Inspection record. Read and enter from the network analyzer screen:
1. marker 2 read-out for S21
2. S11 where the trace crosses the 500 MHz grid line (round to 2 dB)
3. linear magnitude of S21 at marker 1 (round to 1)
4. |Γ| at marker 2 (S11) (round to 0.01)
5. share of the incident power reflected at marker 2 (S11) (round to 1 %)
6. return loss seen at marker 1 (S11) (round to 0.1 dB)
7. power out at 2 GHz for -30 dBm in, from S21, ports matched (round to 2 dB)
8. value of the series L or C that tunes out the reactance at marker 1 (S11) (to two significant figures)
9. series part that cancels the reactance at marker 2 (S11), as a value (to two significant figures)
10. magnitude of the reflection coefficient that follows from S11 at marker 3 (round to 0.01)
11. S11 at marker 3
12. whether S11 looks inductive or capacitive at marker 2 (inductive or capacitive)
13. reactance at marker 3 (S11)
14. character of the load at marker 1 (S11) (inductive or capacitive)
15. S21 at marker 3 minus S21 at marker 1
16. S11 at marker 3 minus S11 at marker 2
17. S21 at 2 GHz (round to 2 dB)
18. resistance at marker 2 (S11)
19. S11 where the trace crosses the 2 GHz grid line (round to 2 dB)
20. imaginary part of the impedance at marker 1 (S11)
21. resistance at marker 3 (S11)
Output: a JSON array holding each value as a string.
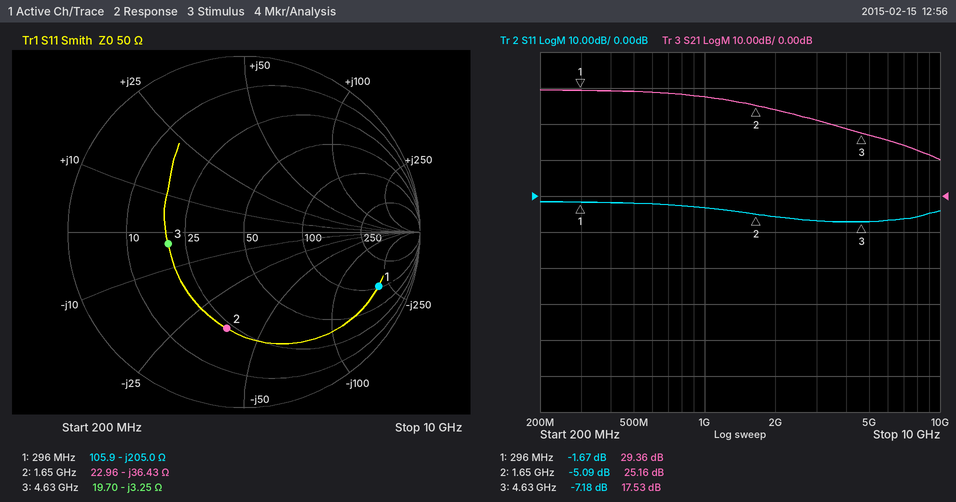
["25.16 dB", "-2 dB", "29", "0.56", "31 %", "1.7 dB", "-6 dBm", "110 nH", "3.5 nH", "0.44", "-7.18 dB", "capacitive", "-3.25 Ω", "capacitive", "-11.83 dB", "-2.09 dB", "24 dB", "22.96 Ω", "-6 dB", "-205.0 Ω", "19.70 Ω"]
